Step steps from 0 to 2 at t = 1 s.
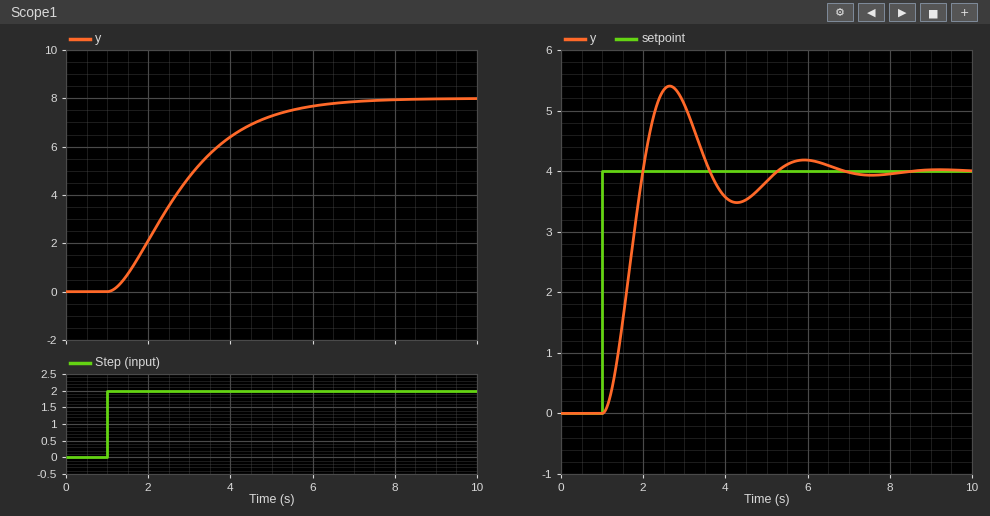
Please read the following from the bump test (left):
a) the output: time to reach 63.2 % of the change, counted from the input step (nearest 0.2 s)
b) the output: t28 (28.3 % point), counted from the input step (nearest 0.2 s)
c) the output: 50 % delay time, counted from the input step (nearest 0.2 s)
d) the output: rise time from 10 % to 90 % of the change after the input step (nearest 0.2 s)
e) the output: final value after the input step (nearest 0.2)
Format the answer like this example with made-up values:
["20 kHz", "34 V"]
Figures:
["2.2 s", "1.0 s", "1.6 s", "3.4 s", "8.0"]
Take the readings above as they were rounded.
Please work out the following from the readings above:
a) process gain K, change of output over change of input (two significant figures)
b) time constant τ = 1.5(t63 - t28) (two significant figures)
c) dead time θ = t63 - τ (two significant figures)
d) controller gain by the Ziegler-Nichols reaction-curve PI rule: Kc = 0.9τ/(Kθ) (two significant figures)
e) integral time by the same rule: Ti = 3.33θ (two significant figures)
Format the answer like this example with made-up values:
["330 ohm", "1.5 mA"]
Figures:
["4.0", "1.8 s", "0.40 s", "1.0", "1.3 s"]
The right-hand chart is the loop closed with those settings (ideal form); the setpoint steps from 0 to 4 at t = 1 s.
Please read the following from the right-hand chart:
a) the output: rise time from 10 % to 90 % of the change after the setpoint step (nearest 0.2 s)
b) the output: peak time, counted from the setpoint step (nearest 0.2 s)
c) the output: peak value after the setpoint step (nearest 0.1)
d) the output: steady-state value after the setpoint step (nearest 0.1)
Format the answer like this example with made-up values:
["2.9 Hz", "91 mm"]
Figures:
["0.6 s", "1.6 s", "5.4", "4.0"]
